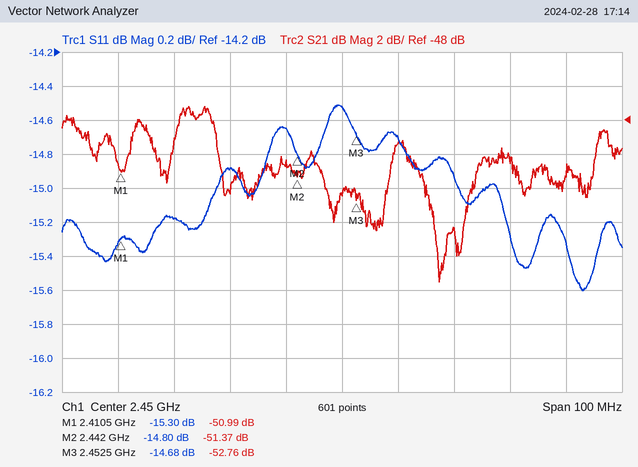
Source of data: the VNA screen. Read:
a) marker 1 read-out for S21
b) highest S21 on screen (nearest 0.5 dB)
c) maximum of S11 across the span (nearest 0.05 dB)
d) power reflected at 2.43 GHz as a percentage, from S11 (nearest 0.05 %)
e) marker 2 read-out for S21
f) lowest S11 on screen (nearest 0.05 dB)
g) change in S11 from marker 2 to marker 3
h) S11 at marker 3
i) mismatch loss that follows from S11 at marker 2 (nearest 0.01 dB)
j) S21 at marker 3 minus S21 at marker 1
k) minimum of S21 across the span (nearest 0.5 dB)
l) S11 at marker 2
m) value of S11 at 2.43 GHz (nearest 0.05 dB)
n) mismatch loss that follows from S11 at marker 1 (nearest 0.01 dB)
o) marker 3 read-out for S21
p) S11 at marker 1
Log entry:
-50.99 dB
-47.0 dB
-14.50 dB
3.25 %
-51.37 dB
-15.60 dB
0.12 dB
-14.68 dB
0.15 dB
-1.77 dB
-57.5 dB
-14.80 dB
-14.90 dB
0.13 dB
-52.76 dB
-15.30 dB
